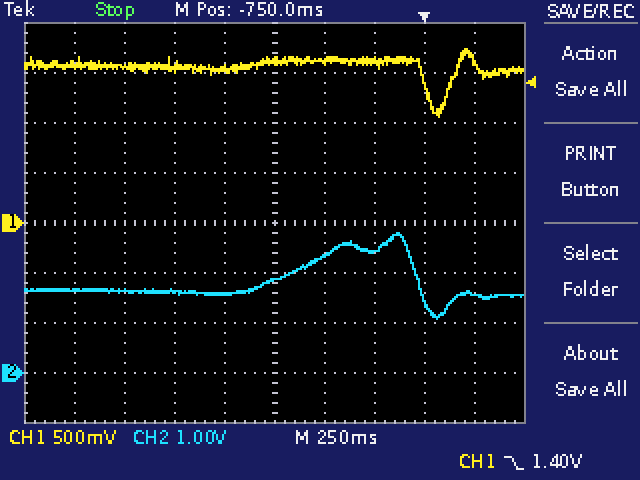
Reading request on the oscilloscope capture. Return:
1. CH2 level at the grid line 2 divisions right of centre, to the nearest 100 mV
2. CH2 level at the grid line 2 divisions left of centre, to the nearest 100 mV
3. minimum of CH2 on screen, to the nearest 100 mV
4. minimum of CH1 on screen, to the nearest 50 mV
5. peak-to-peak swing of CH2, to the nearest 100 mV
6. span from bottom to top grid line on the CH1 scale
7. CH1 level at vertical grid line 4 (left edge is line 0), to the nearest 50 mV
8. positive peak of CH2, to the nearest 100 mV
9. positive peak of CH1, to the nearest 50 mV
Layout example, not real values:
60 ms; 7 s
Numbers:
2.4 V; 1.6 V; 1.1 V; 1.05 V; 1.7 V; 4 V; 1.55 V; 2.8 V; 1.75 V
